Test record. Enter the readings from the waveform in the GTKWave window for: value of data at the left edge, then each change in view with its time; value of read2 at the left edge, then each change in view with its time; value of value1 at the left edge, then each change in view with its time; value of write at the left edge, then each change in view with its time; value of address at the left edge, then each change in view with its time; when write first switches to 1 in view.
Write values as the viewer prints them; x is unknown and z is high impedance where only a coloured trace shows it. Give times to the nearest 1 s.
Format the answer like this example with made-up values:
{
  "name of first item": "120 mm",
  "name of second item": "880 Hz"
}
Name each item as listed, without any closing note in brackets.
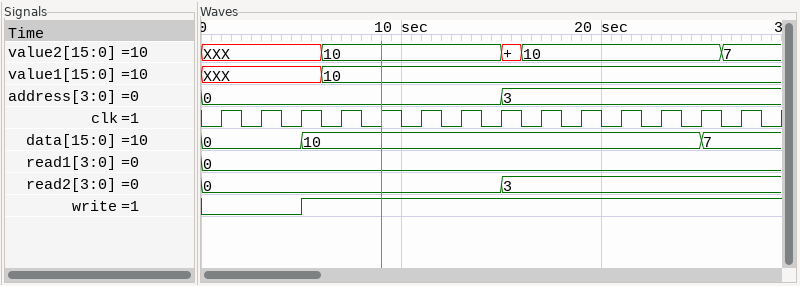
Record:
{
  "value of data at the left edge, then each change in view with its time": "0, 10 at 5 s, 7 at 25 s",
  "value of read2 at the left edge, then each change in view with its time": "0, 3 at 15 s",
  "value of value1 at the left edge, then each change in view with its time": "XXX, 10 at 6 s",
  "value of write at the left edge, then each change in view with its time": "0, 1 at 5 s",
  "value of address at the left edge, then each change in view with its time": "0, 3 at 15 s",
  "when write first switches to 1 in view": "5 s"
}
